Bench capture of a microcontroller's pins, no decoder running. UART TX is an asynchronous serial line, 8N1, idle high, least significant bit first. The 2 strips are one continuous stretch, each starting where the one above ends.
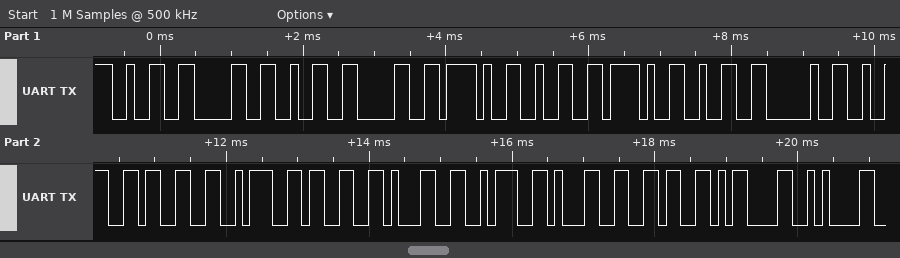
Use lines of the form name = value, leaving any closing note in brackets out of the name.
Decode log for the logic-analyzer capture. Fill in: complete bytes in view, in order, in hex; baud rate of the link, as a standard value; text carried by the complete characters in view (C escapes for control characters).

complete bytes in view, in order, in hex = 0x32 0x30 0x32 0x30 0x2F 0x32 0x2F 0x32 0x20 0x32 0x33 0x3A 0x33 0x31 0x3A 0x31 0x36 0x0D 0x0A
baud rate of the link, as a standard value = 9600 baud
text carried by the complete characters in view = "2020/2/2 23:31:16\r\n"
